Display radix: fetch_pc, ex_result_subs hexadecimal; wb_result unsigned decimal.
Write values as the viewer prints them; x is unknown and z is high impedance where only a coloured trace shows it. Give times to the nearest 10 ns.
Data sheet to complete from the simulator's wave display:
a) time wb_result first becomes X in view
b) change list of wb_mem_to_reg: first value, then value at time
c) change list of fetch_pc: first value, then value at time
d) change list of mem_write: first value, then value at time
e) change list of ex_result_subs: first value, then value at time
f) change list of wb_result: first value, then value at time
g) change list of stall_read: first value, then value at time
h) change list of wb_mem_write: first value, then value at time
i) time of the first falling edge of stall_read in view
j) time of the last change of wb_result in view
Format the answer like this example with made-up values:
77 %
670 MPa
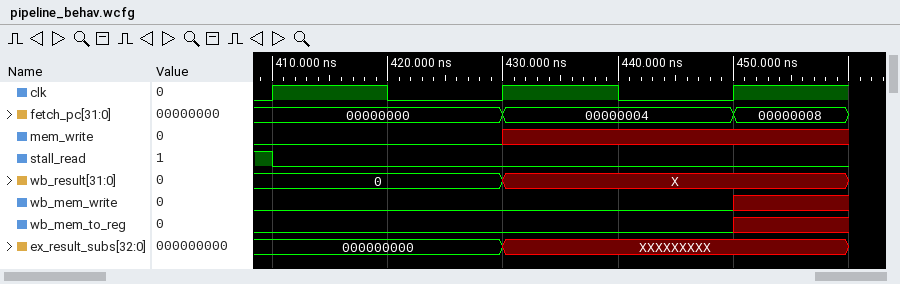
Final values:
430 ns
0, x at 450 ns
00000000, 00000004 at 430 ns, 00000008 at 450 ns
0, x at 430 ns
000000000, XXXXXXXXX at 430 ns
0, X at 430 ns
1, 0 at 410 ns
0, x at 450 ns
410 ns
430 ns
